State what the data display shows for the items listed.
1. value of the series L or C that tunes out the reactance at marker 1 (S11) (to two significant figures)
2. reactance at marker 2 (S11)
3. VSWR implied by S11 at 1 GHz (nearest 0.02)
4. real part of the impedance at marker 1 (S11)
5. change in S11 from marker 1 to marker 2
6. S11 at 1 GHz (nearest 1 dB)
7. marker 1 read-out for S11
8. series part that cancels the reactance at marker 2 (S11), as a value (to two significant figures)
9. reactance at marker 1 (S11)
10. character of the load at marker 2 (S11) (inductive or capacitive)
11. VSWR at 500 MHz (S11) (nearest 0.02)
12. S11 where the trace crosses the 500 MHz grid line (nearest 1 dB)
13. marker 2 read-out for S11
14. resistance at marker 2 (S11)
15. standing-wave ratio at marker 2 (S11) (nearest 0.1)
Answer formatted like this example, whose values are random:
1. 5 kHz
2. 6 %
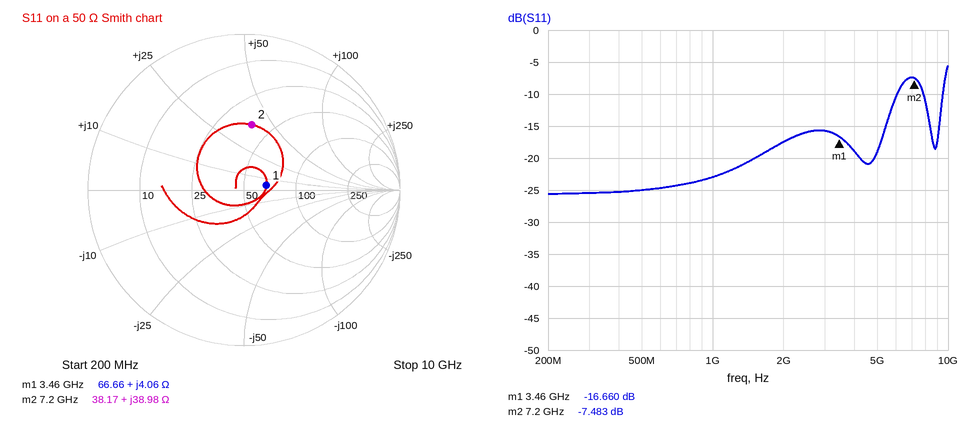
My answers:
1. 11 pF
2. +38.98 Ω
3. 1.16
4. 66.66 Ω
5. 9.177 dB
6. -23 dB
7. -16.660 dB
8. 570 fF
9. +4.06 Ω
10. inductive
11. 1.12
12. -25 dB
13. -7.483 dB
14. 38.17 Ω
15. 2.5
